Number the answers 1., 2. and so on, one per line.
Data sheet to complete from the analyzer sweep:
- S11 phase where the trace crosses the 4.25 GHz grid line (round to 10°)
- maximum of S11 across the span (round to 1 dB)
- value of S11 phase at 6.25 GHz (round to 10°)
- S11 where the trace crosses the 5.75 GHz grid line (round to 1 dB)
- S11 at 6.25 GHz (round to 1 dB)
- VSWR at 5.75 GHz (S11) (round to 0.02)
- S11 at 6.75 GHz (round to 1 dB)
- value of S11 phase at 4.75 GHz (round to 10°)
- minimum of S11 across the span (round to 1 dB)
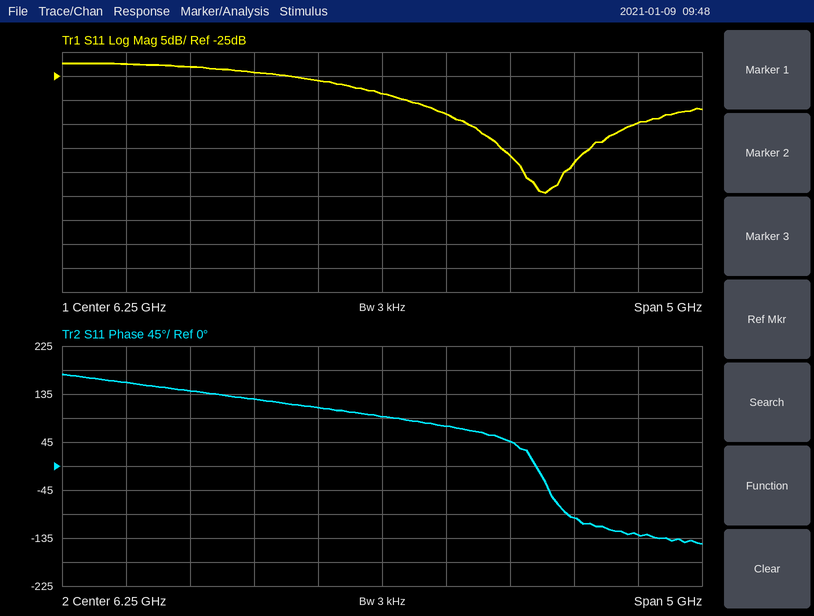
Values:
1. 160°
2. -22 dB
3. 90°
4. -26 dB
5. -29 dB
6. 1.10
7. -33 dB
8. 140°
9. -49 dB
